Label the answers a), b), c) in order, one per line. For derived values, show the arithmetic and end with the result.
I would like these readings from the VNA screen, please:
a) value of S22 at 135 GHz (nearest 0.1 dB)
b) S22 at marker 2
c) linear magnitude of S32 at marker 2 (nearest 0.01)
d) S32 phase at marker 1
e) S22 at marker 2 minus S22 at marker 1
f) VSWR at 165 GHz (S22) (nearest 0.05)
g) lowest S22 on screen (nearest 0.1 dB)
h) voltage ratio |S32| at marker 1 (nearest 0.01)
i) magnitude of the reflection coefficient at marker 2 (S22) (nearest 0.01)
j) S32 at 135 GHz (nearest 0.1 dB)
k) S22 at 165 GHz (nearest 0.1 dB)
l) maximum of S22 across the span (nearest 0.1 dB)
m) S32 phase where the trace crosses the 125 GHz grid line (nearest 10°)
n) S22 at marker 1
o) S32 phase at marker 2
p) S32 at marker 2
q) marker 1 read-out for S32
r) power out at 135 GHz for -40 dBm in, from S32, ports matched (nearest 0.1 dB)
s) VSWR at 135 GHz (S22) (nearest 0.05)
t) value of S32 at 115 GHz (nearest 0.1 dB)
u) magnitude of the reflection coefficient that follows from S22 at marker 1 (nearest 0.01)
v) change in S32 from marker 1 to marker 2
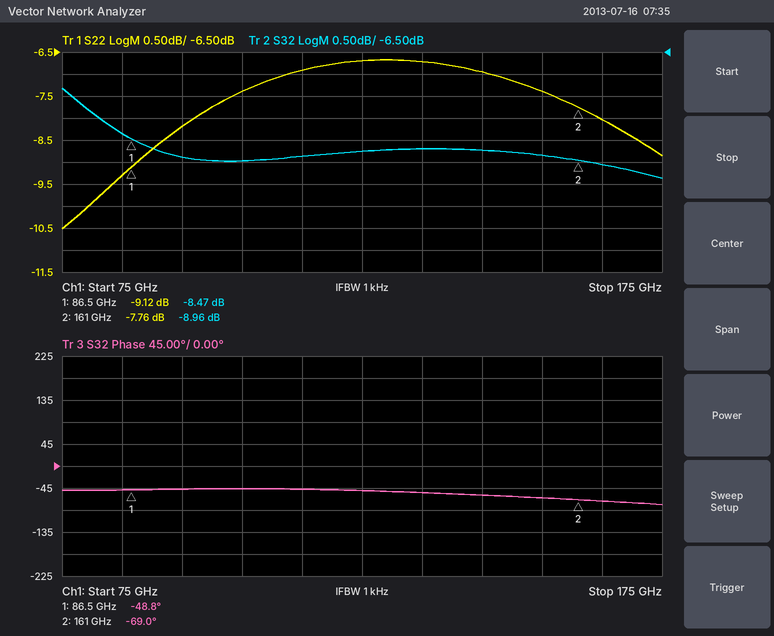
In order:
a) -6.7 dB
b) -7.76 dB
c) 10^(-8.96/20) ≈ 0.36
d) -48.8°
e) -7.76 − (-9.12) = 1.36 dB
f) |Γ| = 10^(-8/20) = 0.3981; VSWR = (1 + 0.3981)/(1 − 0.3981) ≈ 2.32, so 2.30 to the nearest 0.05
g) -10.5 dB
h) 10^(-8.47/20) ≈ 0.38
i) 10^(-7.76/20) ≈ 0.41
j) -8.7 dB
k) -8.0 dB
l) -6.7 dB
m) -50°
n) -9.12 dB
o) -69.0°
p) -8.96 dB
q) -8.47 dB
r) -40 dBm + (-8.7 dB) = -48.7 dBm
s) |Γ| = 10^(-6.7/20) = 0.4624; VSWR = (1 + 0.4624)/(1 − 0.4624) ≈ 2.72, so 2.70 to the nearest 0.05
t) -8.9 dB
u) 10^(-9.12/20) ≈ 0.35
v) -8.96 − (-8.47) = -0.49 dB
